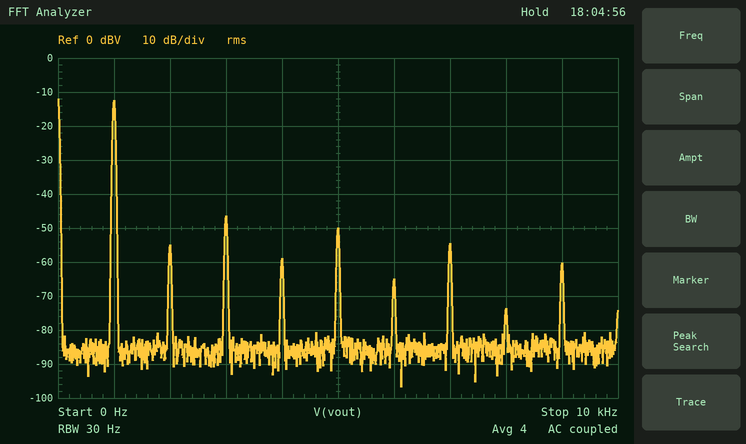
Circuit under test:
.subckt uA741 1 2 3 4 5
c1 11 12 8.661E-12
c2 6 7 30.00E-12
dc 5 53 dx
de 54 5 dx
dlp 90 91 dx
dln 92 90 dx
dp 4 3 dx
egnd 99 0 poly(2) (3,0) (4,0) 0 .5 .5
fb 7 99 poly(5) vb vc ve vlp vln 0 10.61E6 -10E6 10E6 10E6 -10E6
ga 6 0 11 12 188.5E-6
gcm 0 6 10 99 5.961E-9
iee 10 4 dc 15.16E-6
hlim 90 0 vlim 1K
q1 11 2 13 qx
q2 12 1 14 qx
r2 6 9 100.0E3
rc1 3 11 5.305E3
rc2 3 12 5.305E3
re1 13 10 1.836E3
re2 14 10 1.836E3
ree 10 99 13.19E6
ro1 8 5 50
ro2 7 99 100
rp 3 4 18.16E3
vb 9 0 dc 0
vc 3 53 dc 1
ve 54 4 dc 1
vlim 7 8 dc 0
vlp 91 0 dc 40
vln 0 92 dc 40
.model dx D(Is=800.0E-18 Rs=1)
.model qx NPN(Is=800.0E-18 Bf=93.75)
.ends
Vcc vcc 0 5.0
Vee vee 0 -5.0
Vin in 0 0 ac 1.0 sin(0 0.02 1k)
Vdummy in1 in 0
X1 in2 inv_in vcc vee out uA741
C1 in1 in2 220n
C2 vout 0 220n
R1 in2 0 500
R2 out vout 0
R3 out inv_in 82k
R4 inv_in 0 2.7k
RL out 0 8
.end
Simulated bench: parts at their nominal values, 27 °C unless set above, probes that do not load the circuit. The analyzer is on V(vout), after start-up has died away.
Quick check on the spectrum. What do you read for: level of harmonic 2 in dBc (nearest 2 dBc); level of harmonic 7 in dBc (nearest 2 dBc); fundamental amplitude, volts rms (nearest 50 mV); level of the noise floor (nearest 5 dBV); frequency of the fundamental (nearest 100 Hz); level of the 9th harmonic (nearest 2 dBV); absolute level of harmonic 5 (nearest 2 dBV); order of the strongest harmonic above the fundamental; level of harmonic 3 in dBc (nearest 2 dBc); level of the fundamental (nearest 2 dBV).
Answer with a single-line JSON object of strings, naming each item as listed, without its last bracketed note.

{"level of harmonic 2 in dBc": "-42 dBc", "level of harmonic 7 in dBc": "-42 dBc", "fundamental amplitude, volts rms": "250 mV", "level of the noise floor": "-85 dBV", "frequency of the fundamental": "1.0 kHz", "level of the 9th harmonic": "-60 dBV", "absolute level of harmonic 5": "-50 dBV", "order of the strongest harmonic above the fundamental": "3", "level of harmonic 3 in dBc": "-34 dBc", "level of the fundamental": "-12 dBV"}
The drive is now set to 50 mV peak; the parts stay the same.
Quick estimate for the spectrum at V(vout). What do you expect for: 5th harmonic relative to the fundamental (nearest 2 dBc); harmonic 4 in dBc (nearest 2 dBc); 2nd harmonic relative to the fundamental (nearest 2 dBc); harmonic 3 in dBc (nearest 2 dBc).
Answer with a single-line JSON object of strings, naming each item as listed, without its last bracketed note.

{"5th harmonic relative to the fundamental": "-22 dBc", "harmonic 4 in dBc": "-48 dBc", "2nd harmonic relative to the fundamental": "-44 dBc", "harmonic 3 in dBc": "-12 dBc"}
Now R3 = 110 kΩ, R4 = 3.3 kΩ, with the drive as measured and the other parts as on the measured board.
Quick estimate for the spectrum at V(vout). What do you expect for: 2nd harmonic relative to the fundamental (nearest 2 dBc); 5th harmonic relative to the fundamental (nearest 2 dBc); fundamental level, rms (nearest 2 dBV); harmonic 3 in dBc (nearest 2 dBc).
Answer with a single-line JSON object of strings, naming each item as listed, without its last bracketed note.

{"2nd harmonic relative to the fundamental": "-38 dBc", "5th harmonic relative to the fundamental": "-32 dBc", "fundamental level, rms": "-12 dBV", "harmonic 3 in dBc": "-26 dBc"}
